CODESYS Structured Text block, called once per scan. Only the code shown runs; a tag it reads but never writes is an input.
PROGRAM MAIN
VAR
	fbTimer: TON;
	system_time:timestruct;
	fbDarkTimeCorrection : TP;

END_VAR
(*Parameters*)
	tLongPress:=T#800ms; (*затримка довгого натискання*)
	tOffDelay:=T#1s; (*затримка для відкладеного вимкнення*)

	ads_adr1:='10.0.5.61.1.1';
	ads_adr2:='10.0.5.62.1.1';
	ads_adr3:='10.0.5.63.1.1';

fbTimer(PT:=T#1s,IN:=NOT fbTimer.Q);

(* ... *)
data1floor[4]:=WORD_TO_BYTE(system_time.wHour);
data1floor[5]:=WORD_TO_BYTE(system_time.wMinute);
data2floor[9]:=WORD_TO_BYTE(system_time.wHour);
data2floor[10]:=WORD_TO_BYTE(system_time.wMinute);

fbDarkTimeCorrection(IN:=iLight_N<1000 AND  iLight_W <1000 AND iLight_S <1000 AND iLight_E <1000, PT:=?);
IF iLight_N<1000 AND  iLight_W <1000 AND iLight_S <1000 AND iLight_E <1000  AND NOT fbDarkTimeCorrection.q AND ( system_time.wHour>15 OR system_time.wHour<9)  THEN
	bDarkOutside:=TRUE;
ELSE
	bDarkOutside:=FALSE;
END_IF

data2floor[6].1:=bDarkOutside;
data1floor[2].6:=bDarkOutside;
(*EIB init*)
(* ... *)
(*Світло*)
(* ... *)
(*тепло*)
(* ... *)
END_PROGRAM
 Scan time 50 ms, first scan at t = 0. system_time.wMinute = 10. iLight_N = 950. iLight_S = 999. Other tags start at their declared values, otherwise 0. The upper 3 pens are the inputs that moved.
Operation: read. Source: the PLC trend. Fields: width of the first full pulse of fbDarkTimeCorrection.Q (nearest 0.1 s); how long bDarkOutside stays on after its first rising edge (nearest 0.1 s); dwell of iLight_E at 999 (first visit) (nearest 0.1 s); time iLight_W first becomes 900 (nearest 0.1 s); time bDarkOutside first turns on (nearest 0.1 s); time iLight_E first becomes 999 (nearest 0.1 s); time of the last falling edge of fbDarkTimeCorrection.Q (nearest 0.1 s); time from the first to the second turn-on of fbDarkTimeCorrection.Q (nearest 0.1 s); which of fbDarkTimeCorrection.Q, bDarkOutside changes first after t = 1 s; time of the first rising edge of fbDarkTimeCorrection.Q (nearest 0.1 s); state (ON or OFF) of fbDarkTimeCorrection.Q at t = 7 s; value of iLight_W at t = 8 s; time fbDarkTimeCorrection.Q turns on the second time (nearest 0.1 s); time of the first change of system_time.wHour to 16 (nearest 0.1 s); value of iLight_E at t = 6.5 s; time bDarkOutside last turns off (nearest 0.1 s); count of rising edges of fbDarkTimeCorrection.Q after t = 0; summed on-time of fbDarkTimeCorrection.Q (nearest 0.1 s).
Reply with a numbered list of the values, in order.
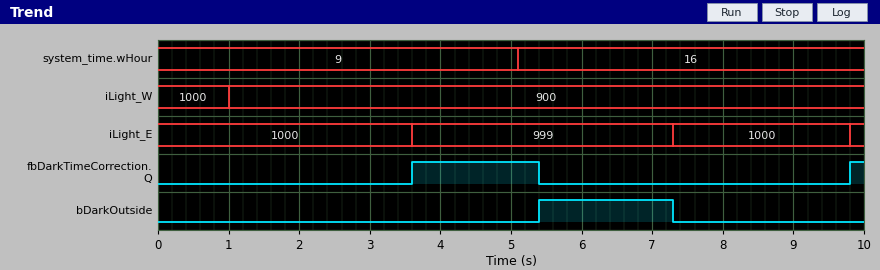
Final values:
1. 1.8 s
2. 1.9 s
3. 3.7 s
4. 1.0 s
5. 5.4 s
6. 3.6 s
7. 5.4 s
8. 6.2 s
9. fbDarkTimeCorrection.Q
10. 3.6 s
11. OFF
12. 900
13. 9.8 s
14. 5.1 s
15. 999
16. 7.3 s
17. 2
18. 2.0 s
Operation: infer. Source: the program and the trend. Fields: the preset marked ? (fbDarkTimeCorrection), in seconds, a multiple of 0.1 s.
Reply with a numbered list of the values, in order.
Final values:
1. 1.8 s
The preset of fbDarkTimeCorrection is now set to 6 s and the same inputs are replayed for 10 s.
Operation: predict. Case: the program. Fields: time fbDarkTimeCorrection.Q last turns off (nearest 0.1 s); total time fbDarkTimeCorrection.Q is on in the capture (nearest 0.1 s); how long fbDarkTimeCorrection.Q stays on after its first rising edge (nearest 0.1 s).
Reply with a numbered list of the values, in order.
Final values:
1. 9.6 s
2. 6.2 s
3. 6.0 s
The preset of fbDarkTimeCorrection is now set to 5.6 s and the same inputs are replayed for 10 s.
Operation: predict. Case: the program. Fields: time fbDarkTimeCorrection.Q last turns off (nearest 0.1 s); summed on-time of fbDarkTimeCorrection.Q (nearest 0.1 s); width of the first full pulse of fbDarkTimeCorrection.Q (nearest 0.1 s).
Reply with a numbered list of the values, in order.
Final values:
1. 9.2 s
2. 5.8 s
3. 5.6 s
